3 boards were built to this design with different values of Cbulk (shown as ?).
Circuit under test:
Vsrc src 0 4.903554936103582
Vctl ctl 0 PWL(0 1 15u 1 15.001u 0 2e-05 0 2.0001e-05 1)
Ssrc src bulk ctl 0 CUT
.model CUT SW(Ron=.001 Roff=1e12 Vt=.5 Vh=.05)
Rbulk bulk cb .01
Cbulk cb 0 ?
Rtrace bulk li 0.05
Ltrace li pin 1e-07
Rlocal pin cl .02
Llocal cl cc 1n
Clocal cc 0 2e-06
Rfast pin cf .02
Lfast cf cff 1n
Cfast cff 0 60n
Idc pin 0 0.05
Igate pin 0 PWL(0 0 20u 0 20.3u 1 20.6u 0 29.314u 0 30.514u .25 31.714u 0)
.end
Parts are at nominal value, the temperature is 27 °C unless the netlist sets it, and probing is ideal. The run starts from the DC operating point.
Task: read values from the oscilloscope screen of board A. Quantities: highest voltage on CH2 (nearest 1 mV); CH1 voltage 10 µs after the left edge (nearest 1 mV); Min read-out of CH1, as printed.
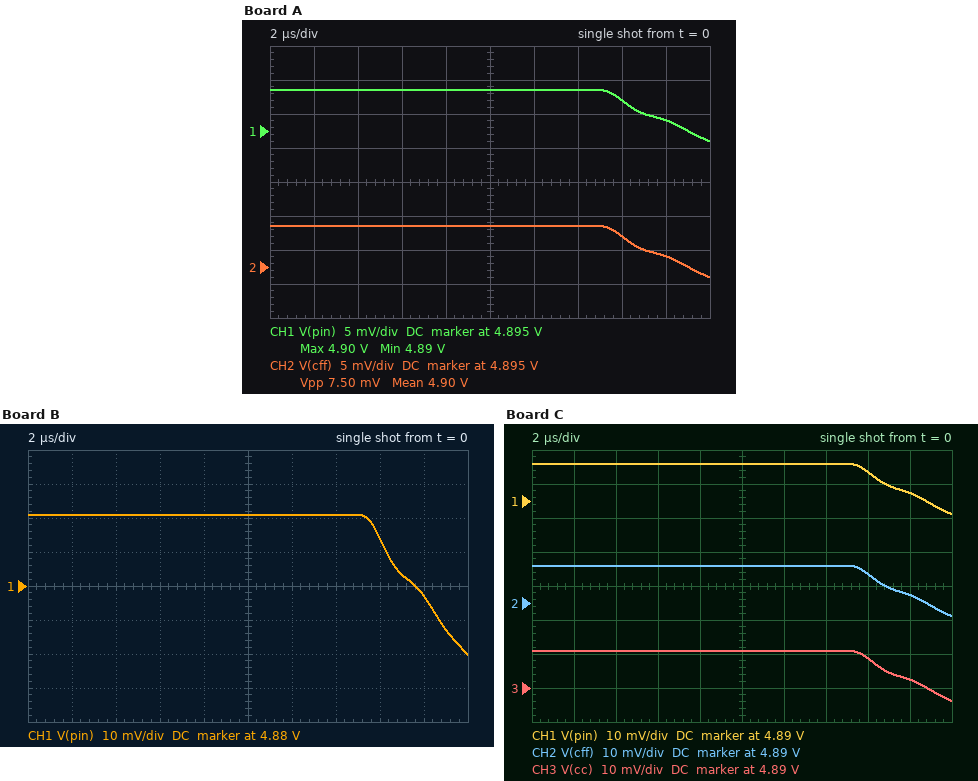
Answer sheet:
4.901 V
4.901 V
4.89 V
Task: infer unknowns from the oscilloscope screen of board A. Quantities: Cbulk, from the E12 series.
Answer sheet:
33 µF
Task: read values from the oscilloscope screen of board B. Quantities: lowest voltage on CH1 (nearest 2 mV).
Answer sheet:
4.860 V
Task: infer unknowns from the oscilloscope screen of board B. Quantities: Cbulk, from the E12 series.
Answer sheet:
3.9 µF
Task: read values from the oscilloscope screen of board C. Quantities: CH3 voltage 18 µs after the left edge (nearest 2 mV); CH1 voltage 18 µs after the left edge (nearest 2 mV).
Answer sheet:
4.892 V
4.892 V
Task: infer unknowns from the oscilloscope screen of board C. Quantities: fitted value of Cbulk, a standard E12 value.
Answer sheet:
15 µF
